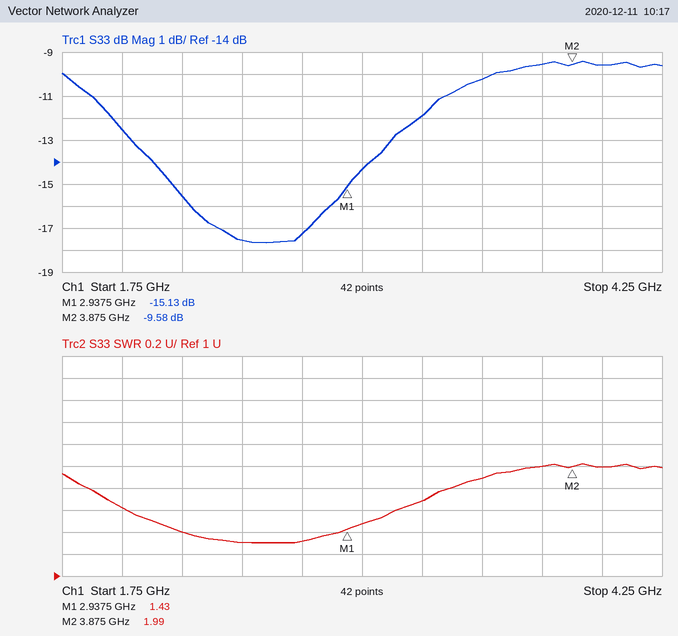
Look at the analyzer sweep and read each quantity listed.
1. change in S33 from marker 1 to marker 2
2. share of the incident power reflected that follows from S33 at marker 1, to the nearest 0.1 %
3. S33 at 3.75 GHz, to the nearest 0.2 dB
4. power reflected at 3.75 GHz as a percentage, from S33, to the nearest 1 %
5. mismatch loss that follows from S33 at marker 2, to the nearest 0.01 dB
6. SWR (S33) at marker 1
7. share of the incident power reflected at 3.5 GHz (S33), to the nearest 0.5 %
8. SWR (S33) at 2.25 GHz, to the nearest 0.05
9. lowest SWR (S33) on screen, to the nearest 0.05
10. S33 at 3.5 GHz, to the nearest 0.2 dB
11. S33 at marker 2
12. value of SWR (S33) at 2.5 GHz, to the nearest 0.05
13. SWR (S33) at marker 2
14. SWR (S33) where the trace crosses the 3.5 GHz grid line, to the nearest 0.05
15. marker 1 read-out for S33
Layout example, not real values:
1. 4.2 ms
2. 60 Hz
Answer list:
1. 5.55 dB
2. 3.1 %
3. -9.6 dB
4. 11 %
5. 0.51 dB
6. 1.43
7. 9.5 %
8. 1.40
9. 1.30
10. -10.2 dB
11. -9.58 dB
12. 1.30
13. 1.99
14. 1.90
15. -15.13 dB
